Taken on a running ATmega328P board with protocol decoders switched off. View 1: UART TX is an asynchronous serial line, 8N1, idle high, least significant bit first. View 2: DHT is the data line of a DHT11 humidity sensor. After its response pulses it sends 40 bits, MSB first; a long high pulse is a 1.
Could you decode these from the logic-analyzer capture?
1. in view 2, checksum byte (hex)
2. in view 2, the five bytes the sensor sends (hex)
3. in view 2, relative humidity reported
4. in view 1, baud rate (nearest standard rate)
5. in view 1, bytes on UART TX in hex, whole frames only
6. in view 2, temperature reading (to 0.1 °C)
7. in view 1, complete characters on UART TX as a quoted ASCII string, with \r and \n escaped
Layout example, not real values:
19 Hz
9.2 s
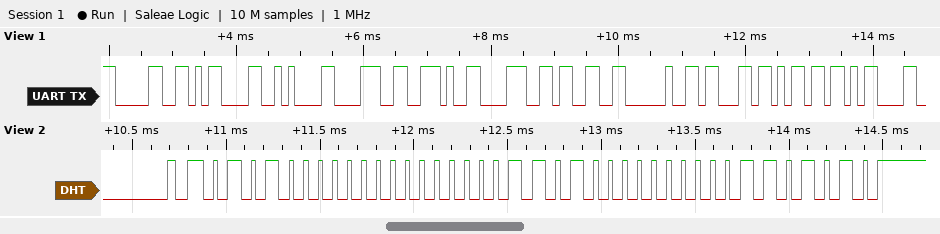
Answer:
0x6A
50 00 1A 00 6A
80 %
9600 baud
0x30 0x0D 0x0A 0x38 0x2E 0x38 0x33 0x20 0x63 0x6D 0x0D
26.0 °C
"0\r\n8.83 cm\r"
